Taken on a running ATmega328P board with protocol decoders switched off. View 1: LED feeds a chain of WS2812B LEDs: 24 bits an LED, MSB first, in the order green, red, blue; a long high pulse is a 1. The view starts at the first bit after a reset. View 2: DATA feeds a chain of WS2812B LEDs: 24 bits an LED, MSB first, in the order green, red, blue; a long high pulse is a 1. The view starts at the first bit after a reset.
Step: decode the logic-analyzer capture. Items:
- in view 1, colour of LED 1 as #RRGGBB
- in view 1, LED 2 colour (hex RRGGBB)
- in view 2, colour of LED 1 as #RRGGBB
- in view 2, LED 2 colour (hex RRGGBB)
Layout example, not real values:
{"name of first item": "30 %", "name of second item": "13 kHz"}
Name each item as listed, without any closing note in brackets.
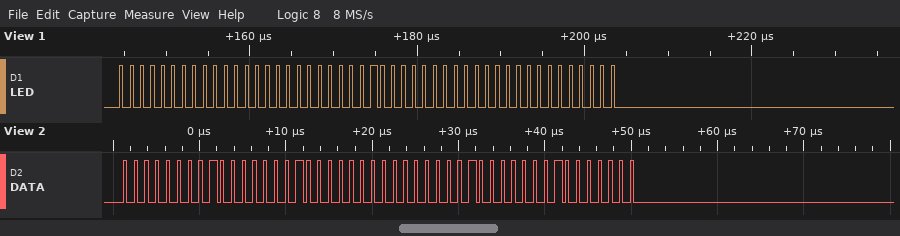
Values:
{"in view 1, colour of LED 1 as #RRGGBB": "#000000", "in view 1, LED 2 colour": "#008000", "in view 2, colour of LED 1 as #RRGGBB": "#800080", "in view 2, LED 2 colour": "#800080"}
